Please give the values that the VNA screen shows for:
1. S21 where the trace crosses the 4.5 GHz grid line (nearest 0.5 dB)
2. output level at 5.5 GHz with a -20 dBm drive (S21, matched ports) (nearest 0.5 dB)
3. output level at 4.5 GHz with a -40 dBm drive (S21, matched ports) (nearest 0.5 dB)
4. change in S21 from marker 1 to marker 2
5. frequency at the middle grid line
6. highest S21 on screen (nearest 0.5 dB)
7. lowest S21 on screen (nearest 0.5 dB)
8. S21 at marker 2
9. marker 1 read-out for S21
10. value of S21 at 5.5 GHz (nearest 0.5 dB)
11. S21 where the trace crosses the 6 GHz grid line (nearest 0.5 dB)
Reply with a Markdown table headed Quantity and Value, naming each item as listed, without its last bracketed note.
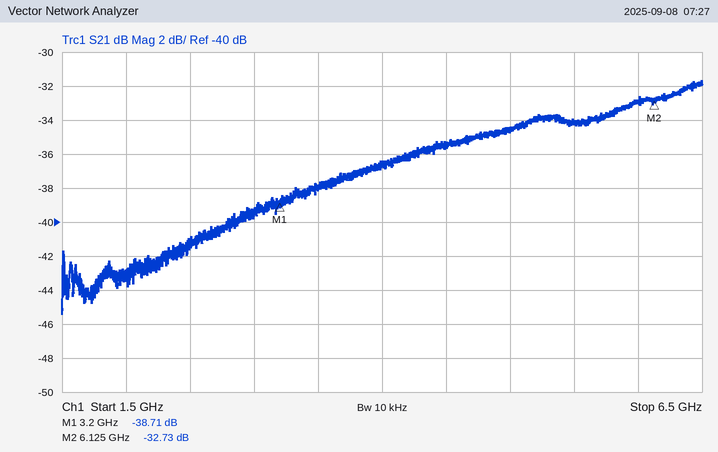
| Quantity | Value |
|---|---|
| S21 where the trace crosses the 4.5 GHz grid line | -35.5 dB |
| output level at 5.5 GHz with a -20 dBm drive (S21, matched ports) | -54.0 dBm |
| output level at 4.5 GHz with a -40 dBm drive (S21, matched ports) | -75.5 dBm |
| change in S21 from marker 1 to marker 2 | 5.98 dB |
| frequency at the middle grid line | 4 GHz |
| highest S21 on screen | -31.5 dB |
| lowest S21 on screen | -45.5 dB |
| S21 at marker 2 | -32.73 dB |
| marker 1 read-out for S21 | -38.71 dB |
| value of S21 at 5.5 GHz | -34.0 dB |
| S21 where the trace crosses the 6 GHz grid line | -33.0 dB |
